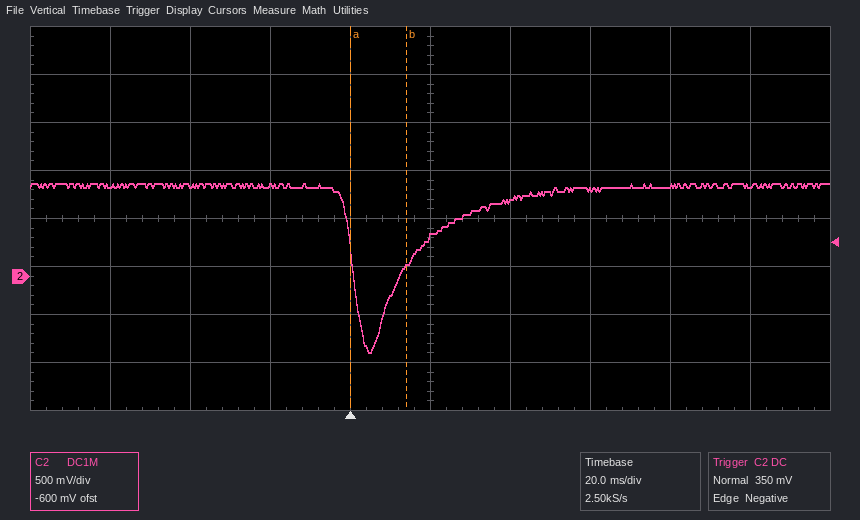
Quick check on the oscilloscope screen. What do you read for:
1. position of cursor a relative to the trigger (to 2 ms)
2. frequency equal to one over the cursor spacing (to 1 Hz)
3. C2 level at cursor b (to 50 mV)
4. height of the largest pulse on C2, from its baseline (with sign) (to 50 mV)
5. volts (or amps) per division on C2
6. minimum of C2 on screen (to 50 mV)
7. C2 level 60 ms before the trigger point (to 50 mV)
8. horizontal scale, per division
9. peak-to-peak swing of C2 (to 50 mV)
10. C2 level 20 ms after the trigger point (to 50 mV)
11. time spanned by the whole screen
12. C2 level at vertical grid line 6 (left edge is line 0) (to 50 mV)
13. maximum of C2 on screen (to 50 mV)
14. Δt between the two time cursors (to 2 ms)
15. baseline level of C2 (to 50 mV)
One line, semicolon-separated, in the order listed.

0 ms; 71 Hz; 100 mV; -1.75 V; 500 mV; -800 mV; 950 mV; 20 ms; 1.75 V; 400 mV; 200 ms; 800 mV; 950 mV; 14 ms; 950 mV
